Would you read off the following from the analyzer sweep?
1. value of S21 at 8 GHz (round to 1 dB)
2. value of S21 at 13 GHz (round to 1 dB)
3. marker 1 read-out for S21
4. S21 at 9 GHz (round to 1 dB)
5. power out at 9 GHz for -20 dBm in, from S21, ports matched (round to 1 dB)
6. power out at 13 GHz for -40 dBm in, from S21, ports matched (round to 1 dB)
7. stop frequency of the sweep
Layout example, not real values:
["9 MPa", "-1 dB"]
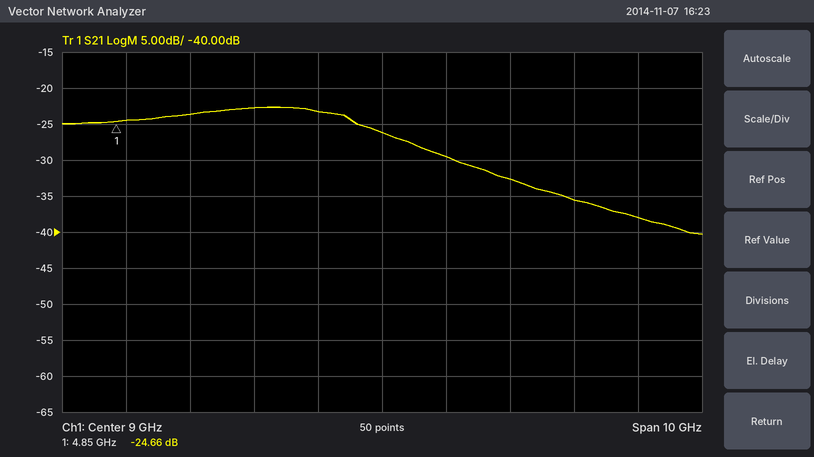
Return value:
["-23 dB", "-38 dB", "-24.66 dB", "-26 dB", "-46 dBm", "-78 dBm", "14 GHz"]
